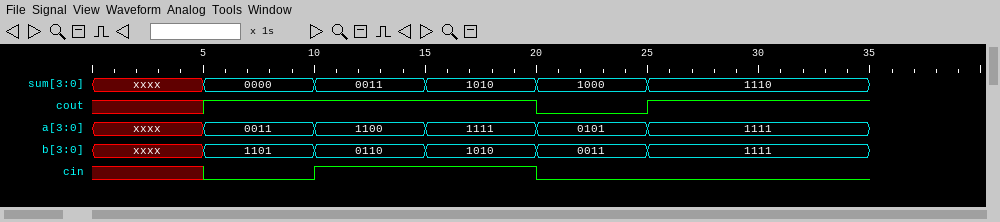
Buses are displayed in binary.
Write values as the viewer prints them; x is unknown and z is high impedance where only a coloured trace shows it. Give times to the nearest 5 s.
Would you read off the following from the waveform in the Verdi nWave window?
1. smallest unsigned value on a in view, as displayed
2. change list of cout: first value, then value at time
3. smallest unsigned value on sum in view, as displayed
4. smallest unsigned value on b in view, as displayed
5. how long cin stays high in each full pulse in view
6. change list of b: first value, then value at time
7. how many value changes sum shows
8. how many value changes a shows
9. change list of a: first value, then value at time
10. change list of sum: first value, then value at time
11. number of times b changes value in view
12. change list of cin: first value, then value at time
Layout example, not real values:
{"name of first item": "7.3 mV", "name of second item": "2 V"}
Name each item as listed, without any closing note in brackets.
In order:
{"smallest unsigned value on a in view, as displayed": "0011", "change list of cout: first value, then value at time": "x, 1 at 5 s, 0 at 20 s, 1 at 25 s", "smallest unsigned value on sum in view, as displayed": "0000", "smallest unsigned value on b in view, as displayed": "0011", "how long cin stays high in each full pulse in view": "10 s", "change list of b: first value, then value at time": "xxxx, 1101 at 5 s, 0110 at 10 s, 1010 at 15 s, 0011 at 20 s, 1111 at 25 s", "how many value changes sum shows": "5", "how many value changes a shows": "5", "change list of a: first value, then value at time": "xxxx, 0011 at 5 s, 1100 at 10 s, 1111 at 15 s, 0101 at 20 s, 1111 at 25 s", "change list of sum: first value, then value at time": "xxxx, 0000 at 5 s, 0011 at 10 s, 1010 at 15 s, 1000 at 20 s, 1110 at 25 s", "number of times b changes value in view": "5", "change list of cin: first value, then value at time": "x, 0 at 5 s, 1 at 10 s, 0 at 20 s"}
